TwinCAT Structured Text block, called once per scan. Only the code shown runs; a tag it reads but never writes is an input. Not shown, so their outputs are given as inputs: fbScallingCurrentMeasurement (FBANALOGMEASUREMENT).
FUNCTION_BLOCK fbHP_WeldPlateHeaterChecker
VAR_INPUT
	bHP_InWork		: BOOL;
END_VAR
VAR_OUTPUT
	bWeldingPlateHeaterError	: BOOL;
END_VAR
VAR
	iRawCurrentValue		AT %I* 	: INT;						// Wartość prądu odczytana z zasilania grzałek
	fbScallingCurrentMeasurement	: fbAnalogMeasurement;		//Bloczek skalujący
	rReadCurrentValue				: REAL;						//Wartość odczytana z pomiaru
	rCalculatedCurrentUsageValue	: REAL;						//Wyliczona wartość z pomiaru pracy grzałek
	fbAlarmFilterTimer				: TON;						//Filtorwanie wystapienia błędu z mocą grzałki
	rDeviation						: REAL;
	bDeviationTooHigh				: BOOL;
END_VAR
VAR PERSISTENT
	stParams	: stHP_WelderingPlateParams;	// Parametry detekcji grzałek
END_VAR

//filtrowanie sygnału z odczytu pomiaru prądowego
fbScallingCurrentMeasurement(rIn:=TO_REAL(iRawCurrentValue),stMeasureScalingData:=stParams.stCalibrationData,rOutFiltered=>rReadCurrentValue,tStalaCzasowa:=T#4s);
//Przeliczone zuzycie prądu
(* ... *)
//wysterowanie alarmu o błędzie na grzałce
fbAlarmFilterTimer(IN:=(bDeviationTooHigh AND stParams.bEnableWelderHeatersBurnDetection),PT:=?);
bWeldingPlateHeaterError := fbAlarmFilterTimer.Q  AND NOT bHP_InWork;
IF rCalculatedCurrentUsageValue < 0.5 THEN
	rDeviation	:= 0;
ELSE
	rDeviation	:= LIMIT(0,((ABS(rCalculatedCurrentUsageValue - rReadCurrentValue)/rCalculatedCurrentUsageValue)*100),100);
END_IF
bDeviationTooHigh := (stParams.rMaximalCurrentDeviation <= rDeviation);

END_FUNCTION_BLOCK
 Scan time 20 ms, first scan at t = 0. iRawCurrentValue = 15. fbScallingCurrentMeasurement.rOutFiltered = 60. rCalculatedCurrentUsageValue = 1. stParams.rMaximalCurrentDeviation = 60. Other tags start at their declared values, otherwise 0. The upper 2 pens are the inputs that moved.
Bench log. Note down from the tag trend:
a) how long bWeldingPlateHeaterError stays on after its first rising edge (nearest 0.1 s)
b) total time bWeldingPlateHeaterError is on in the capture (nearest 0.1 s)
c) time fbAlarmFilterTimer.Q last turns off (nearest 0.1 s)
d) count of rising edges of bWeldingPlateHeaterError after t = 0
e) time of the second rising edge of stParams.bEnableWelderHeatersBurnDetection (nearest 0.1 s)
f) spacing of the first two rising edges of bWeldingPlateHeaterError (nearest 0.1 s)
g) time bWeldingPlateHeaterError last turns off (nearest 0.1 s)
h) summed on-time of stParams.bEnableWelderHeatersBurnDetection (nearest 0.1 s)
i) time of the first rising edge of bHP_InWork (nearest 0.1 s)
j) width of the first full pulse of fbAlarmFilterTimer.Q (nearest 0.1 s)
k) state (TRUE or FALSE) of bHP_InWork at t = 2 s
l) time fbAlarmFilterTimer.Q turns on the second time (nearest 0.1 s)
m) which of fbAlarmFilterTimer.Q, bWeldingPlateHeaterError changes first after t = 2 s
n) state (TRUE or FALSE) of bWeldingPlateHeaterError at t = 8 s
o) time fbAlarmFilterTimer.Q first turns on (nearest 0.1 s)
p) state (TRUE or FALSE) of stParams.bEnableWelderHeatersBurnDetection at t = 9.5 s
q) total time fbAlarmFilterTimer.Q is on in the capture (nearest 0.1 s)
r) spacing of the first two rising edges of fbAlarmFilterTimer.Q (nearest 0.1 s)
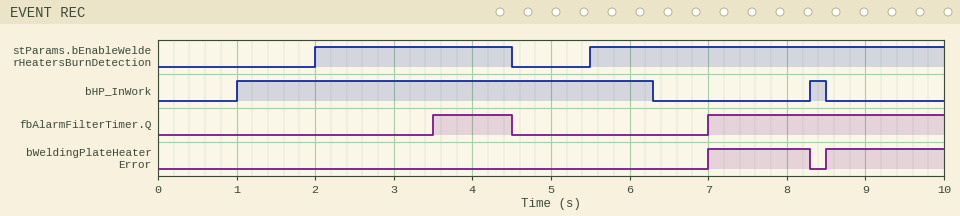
1.3 s
2.8 s
4.5 s
2
5.5 s
1.5 s
8.3 s
7.0 s
1.0 s
1.0 s
TRUE
7.0 s
fbAlarmFilterTimer.Q
TRUE
3.5 s
TRUE
4.0 s
3.5 s
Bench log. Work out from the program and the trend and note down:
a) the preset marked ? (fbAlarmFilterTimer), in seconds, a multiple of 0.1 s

1.5 s
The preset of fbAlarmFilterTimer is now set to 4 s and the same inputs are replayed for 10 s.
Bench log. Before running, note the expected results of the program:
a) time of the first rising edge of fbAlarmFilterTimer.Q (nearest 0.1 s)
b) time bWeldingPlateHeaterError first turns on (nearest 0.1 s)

9.5 s
9.5 s
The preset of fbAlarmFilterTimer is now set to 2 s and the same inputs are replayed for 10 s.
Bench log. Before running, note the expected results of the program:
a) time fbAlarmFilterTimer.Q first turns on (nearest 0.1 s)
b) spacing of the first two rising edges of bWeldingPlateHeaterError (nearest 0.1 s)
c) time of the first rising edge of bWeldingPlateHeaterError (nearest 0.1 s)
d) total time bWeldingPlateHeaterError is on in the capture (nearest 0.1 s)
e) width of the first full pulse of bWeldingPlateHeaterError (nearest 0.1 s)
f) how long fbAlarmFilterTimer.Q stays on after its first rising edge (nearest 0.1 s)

4.0 s
1.0 s
7.5 s
2.3 s
0.8 s
0.5 s
